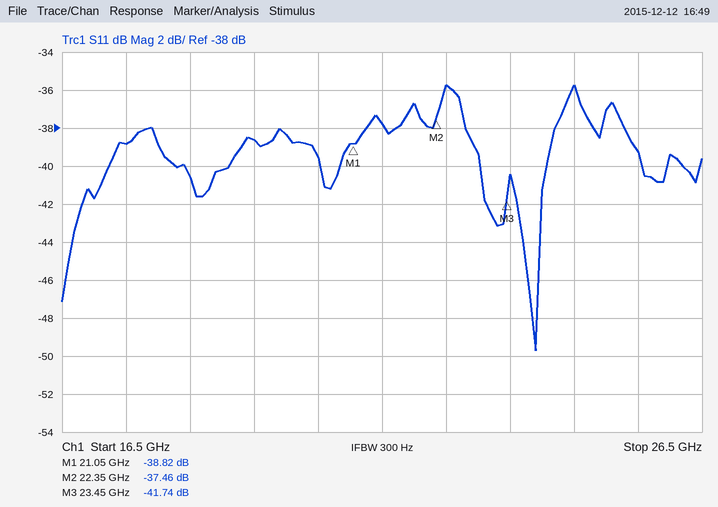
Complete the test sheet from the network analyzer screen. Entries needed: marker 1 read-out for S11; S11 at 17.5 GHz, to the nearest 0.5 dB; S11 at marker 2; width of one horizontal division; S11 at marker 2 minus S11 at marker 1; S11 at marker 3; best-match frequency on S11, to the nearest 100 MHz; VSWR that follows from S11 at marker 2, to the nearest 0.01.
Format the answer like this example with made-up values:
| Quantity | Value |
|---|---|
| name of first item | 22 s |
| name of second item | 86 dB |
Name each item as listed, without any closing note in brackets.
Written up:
| Quantity | Value |
|---|---|
| marker 1 read-out for S11 | -38.82 dB |
| S11 at 17.5 GHz, to the nearest 0.5 dB | -39.0 dB |
| S11 at marker 2 | -37.46 dB |
| width of one horizontal division | 1 GHz |
| S11 at marker 2 minus S11 at marker 1 | 1.36 dB |
| S11 at marker 3 | -41.74 dB |
| best-match frequency on S11, to the nearest 100 MHz | 23.9 GHz |
| VSWR that follows from S11 at marker 2, to the nearest 0.01 | 1.03 |
